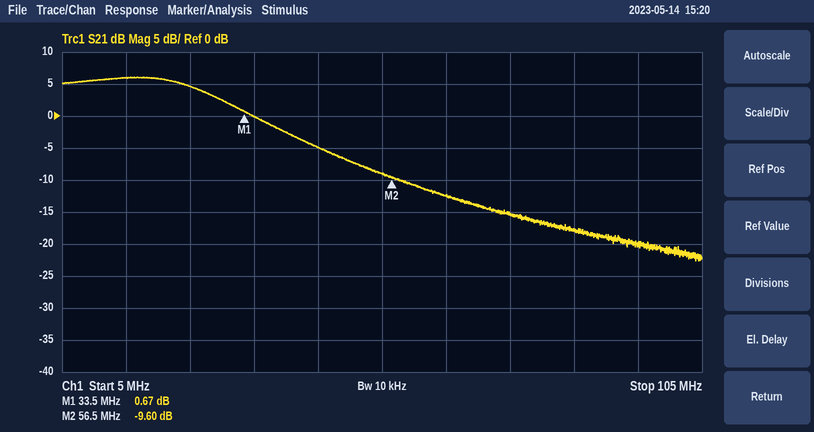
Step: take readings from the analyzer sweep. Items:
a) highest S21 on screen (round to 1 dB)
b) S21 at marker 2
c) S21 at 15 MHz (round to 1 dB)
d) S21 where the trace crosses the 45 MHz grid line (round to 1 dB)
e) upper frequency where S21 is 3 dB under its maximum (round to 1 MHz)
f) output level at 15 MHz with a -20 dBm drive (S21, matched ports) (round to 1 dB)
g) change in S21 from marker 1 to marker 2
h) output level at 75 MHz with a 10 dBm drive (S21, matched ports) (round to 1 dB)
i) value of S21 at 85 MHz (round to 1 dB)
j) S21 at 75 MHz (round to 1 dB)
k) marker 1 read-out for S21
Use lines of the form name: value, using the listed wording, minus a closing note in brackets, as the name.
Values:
highest S21 on screen: 6 dB
S21 at marker 2: -9.60 dB
S21 at 15 MHz: 6 dB
S21 where the trace crosses the 45 MHz grid line: -5 dB
upper frequency where S21 is 3 dB under its maximum: 29 MHz
output level at 15 MHz with a -20 dBm drive (S21, matched ports): -14 dBm
change in S21 from marker 1 to marker 2: -10.27 dB
output level at 75 MHz with a 10 dBm drive (S21, matched ports): -5 dBm
value of S21 at 85 MHz: -18 dB
S21 at 75 MHz: -15 dB
marker 1 read-out for S21: 0.67 dB
